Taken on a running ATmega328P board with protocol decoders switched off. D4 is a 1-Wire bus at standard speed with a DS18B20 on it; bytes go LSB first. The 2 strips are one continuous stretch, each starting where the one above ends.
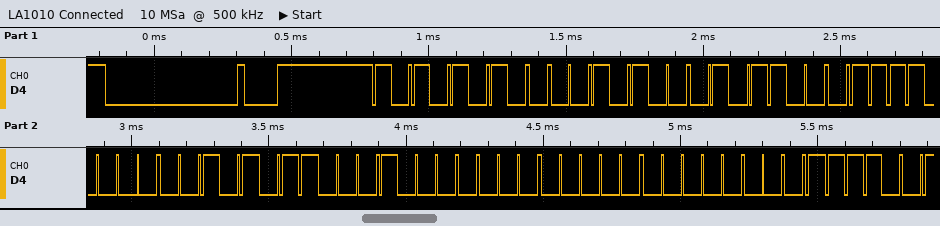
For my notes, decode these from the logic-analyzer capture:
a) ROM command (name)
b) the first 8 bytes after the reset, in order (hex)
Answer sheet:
Match ROM
55 28 1A 0F D4 08 00 00
